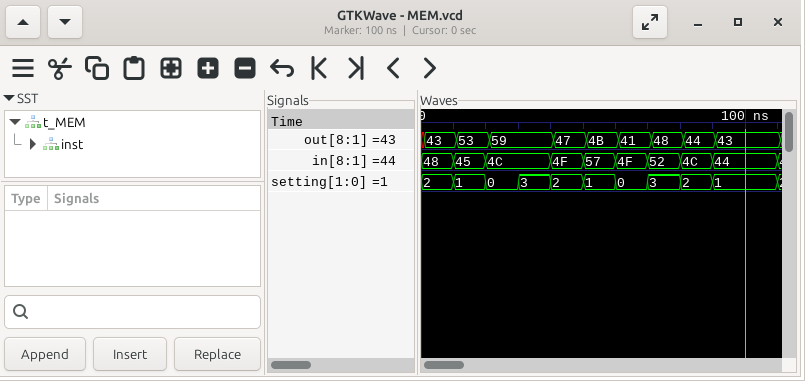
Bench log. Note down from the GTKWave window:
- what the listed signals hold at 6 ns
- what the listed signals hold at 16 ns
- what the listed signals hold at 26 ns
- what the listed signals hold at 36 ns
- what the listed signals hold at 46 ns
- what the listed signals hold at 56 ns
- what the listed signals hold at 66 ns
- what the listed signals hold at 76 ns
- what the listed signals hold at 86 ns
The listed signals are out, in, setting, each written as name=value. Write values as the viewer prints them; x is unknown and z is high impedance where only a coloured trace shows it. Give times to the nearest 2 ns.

out=43, in=48, setting=2
out=53, in=45, setting=1
out=59, in=4C, setting=0
out=59, in=4C, setting=3
out=47, in=4F, setting=2
out=4B, in=57, setting=1
out=41, in=4F, setting=0
out=48, in=52, setting=3
out=44, in=4C, setting=2
